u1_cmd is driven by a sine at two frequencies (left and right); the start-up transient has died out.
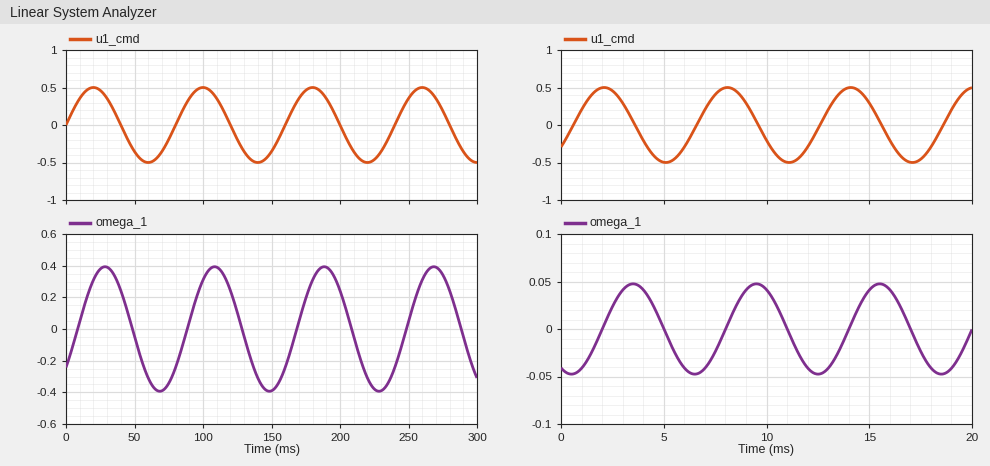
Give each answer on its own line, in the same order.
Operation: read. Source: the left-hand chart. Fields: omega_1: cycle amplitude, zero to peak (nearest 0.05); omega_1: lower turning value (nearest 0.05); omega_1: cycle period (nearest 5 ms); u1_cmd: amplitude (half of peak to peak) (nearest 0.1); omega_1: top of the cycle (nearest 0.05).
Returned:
0.40
-0.40
80 ms
0.5
0.40
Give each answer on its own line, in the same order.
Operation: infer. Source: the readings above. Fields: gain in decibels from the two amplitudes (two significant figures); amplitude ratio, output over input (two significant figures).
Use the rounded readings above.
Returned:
-1.9 dB
0.80
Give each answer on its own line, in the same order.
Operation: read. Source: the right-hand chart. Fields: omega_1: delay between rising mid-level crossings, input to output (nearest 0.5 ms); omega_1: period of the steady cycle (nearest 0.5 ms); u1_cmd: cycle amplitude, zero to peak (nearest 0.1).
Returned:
1.5 ms
6.0 ms
0.5
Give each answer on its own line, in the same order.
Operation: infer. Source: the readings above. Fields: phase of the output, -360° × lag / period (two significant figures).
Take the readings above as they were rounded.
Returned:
-90°
